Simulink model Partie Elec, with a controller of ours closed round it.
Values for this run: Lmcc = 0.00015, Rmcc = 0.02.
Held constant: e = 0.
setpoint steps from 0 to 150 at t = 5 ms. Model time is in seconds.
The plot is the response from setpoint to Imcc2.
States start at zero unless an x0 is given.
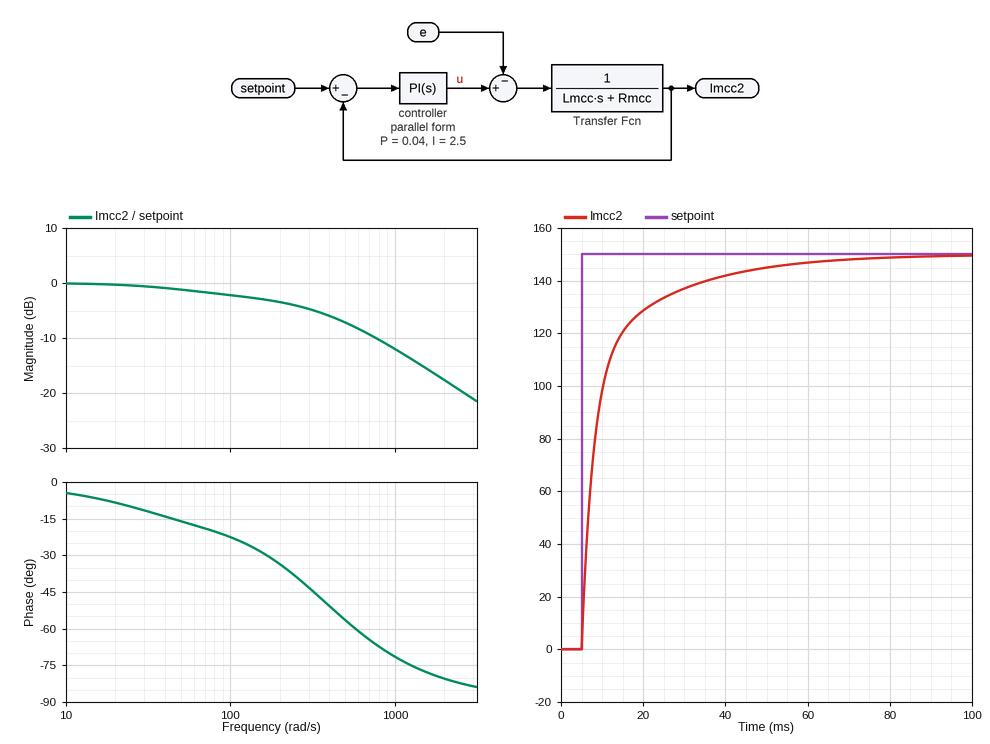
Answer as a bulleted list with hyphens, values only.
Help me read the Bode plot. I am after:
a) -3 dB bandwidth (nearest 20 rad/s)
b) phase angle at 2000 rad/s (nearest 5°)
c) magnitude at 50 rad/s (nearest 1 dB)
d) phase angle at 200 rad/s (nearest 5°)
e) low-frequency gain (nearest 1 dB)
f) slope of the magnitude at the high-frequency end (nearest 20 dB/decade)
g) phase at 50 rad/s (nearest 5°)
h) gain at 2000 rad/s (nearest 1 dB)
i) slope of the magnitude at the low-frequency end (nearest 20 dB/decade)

- 180 rad/s
- -80°
- -1 dB
- -35°
- 0 dB
- -20 dB/decade
- -15°
- -18 dB
- 0 dB/decade
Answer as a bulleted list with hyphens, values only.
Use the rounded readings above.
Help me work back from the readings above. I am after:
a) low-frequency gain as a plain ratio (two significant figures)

- 1.0
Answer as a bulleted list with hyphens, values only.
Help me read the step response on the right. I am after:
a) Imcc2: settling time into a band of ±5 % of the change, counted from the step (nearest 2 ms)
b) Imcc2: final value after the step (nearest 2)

- 36 ms
- 150
